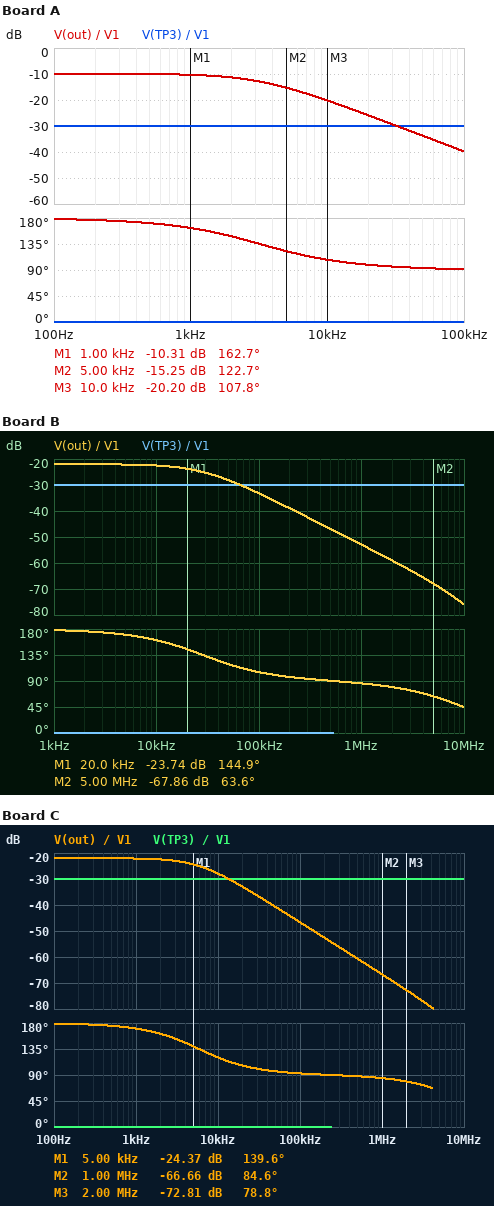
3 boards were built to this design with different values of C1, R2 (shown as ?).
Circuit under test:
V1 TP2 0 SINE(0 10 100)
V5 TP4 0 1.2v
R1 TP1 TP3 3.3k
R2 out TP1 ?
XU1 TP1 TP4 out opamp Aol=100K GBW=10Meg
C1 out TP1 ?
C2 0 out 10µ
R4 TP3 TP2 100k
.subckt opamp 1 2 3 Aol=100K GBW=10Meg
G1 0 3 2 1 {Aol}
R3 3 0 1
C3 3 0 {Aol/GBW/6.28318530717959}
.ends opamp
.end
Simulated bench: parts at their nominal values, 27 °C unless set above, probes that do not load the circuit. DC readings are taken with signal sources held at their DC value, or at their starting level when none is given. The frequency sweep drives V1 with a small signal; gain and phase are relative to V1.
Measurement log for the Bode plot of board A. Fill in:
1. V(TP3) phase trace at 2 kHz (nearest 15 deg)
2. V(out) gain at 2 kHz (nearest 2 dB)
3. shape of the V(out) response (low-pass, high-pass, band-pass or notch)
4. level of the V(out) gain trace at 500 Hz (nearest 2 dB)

0 deg
-12 dB
low-pass
-10 dB
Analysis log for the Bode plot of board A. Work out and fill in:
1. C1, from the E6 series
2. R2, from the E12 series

1.5 nF
33 kΩ
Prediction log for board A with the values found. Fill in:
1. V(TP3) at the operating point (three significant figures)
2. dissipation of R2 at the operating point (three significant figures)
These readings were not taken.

1.16 V
4.45 µW
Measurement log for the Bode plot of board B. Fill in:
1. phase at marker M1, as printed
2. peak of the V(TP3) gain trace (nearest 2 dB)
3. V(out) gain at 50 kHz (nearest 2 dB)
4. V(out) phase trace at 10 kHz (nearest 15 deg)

144.9 deg
-30 dB
-28 dB
165 deg
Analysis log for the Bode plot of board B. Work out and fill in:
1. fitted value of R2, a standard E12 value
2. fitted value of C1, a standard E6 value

8.2 kΩ
680 pF
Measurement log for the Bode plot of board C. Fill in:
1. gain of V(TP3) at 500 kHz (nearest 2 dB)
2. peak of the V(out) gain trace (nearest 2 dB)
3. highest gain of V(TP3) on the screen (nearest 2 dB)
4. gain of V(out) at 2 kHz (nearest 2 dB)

-30 dB
-22 dB
-30 dB
-22 dB
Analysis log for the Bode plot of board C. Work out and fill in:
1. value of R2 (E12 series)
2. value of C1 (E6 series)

8.2 kΩ
3.3 nF
